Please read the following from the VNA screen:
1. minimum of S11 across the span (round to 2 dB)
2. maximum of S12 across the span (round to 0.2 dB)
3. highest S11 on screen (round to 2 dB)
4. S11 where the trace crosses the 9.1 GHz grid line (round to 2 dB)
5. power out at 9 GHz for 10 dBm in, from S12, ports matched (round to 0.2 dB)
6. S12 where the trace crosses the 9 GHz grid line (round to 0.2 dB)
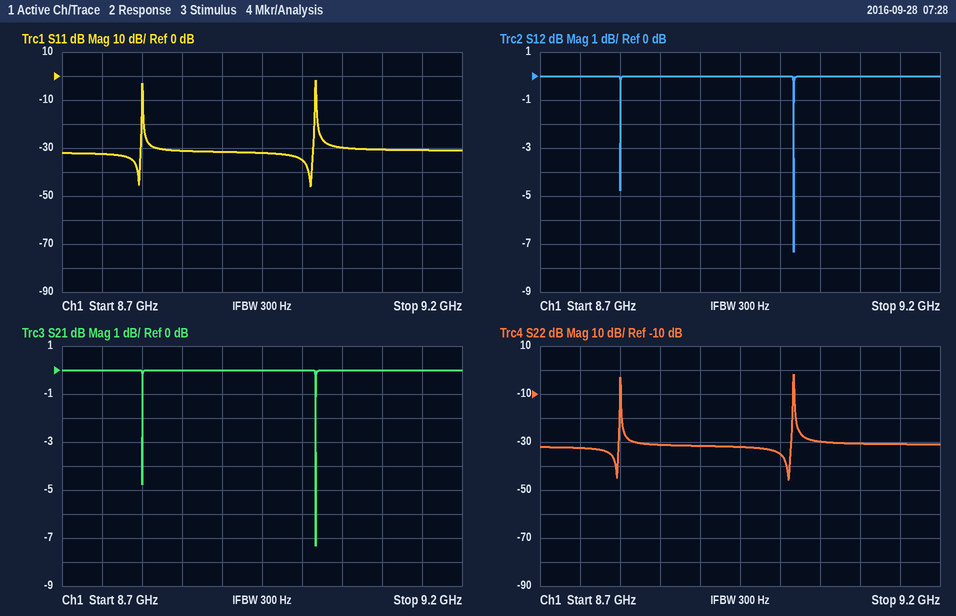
-46 dB
0.0 dB
-2 dB
-30 dB
10.0 dBm
0.0 dB
